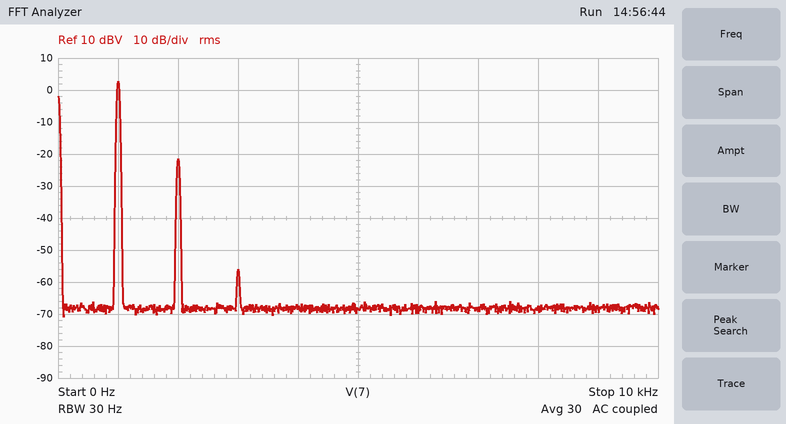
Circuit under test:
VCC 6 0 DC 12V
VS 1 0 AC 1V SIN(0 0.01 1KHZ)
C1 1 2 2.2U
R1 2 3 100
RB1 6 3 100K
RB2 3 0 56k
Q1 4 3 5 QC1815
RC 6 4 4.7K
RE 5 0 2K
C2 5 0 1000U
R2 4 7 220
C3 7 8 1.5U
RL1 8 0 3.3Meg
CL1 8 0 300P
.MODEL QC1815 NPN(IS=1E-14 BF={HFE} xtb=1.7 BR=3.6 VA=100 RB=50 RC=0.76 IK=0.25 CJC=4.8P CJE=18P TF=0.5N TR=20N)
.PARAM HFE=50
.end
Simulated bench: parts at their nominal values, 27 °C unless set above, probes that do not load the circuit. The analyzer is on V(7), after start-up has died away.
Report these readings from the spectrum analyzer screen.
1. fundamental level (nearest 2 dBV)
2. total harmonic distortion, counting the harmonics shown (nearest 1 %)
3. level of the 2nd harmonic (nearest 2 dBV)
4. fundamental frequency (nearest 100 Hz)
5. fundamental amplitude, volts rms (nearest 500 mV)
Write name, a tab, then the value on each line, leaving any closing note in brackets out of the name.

fundamental level	2 dBV
total harmonic distortion, counting the harmonics shown	6 %
level of the 2nd harmonic	-22 dBV
fundamental frequency	1.0 kHz
fundamental amplitude, volts rms	1.5 V
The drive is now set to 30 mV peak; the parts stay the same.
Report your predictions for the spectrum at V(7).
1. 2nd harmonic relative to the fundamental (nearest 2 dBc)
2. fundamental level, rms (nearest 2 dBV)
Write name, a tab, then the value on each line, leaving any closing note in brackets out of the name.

2nd harmonic relative to the fundamental	-20 dBc
fundamental level, rms	10 dBV
